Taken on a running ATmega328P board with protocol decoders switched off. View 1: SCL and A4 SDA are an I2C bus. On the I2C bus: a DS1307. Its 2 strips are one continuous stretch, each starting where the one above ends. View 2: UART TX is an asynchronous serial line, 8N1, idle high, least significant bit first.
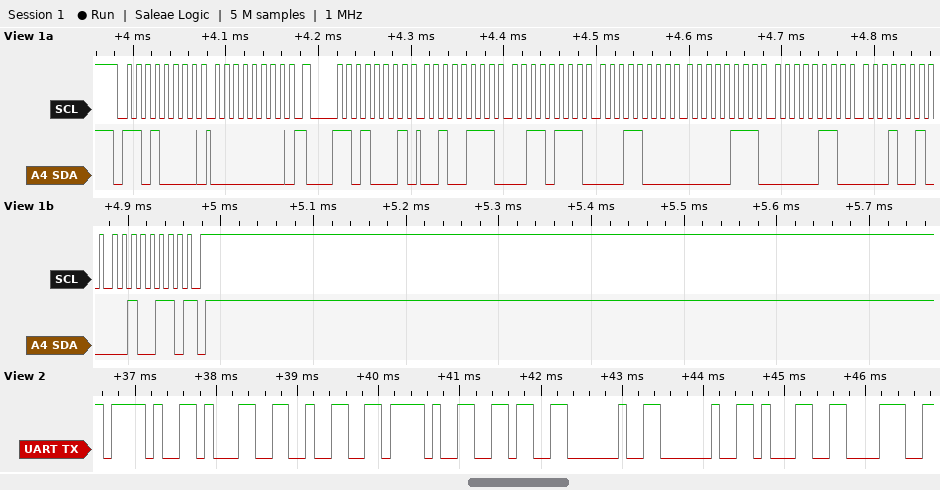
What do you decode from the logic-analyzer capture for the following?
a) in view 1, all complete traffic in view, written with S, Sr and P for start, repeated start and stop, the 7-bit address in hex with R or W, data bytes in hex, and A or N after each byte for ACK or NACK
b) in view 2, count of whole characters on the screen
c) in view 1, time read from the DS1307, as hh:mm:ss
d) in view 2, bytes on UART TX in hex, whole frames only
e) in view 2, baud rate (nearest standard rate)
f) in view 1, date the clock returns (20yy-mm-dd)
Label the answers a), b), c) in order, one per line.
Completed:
a) S 68W A 00 A Sr 68R A 27 A 37 A 18 A 07 A 06 A 12 A 26 N P
b) 9
c) 18:37:27
d) 2F 31 32 2F 36 20 20 31 38
e) 9600 baud
f) 2026-12-06
